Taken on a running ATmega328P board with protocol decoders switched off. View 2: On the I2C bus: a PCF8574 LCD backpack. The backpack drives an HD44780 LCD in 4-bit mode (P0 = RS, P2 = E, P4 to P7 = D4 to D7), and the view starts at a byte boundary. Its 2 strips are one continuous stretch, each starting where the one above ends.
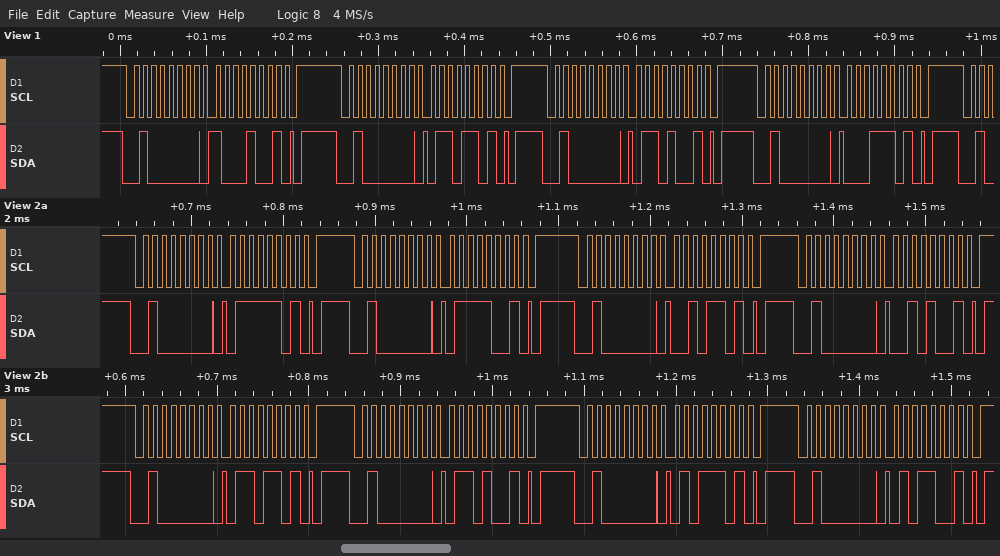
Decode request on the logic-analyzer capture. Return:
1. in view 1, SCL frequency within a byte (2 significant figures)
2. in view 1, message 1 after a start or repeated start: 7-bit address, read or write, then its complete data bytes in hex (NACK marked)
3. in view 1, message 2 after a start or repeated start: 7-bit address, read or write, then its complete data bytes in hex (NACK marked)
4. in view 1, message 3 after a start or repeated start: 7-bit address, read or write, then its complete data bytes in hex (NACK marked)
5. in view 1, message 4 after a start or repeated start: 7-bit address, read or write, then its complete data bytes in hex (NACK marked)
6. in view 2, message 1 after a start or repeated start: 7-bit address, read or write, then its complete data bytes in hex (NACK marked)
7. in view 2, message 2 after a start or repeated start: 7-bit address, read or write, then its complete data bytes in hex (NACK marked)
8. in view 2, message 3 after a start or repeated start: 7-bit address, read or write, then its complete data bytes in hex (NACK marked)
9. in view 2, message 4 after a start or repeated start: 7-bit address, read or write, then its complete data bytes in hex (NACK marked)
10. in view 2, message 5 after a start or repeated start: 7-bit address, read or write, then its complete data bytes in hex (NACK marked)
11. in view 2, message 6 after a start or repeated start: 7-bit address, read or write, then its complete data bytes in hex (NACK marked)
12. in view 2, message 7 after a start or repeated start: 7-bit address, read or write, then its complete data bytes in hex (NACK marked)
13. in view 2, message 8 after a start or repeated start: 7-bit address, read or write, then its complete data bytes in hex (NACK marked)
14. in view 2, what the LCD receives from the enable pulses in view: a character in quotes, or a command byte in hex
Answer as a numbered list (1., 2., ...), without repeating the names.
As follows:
1. 100 kHz
2. 0x20 write: 89
3. 0x20 write: 6D
4. 0x20 write: 69
5. 0x20 write: 1D
6. 0x20 write: 7D
7. 0x20 write: 79
8. 0x20 write: 2D
9. 0x20 write: 29
10. 0x20 write: 6D
11. 0x20 write: 69
12. 0x20 write: 5D
13. 0x20 write: 59
14. 'r' 'e'
